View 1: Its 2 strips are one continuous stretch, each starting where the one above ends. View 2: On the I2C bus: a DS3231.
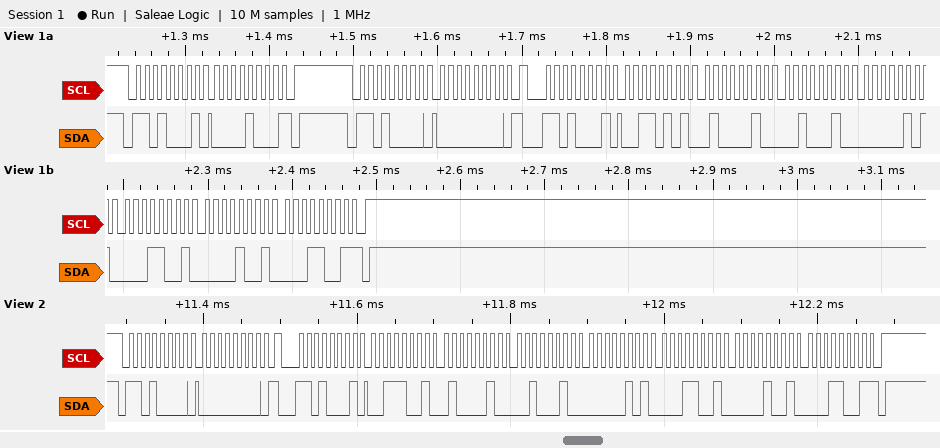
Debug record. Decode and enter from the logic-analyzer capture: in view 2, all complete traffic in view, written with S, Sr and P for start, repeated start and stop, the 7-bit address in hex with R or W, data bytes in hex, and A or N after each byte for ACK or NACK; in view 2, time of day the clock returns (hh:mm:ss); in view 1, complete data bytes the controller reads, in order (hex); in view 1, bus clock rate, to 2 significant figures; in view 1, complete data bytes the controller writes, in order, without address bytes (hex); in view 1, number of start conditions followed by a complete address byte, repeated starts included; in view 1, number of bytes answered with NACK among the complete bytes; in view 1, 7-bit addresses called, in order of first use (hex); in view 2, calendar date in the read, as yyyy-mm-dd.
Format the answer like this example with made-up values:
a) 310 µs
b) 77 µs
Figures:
a) S 68W A 00 A Sr 68R A 39 A 42 A 22 A 05 A 19 A 09 A 19 N P
b) 22:42:39
c) 08 35 42 22 05 19 09 19
d) 100 kHz
e) 00
f) 3
g) 2
h) 0x68
i) 2019-09-19
